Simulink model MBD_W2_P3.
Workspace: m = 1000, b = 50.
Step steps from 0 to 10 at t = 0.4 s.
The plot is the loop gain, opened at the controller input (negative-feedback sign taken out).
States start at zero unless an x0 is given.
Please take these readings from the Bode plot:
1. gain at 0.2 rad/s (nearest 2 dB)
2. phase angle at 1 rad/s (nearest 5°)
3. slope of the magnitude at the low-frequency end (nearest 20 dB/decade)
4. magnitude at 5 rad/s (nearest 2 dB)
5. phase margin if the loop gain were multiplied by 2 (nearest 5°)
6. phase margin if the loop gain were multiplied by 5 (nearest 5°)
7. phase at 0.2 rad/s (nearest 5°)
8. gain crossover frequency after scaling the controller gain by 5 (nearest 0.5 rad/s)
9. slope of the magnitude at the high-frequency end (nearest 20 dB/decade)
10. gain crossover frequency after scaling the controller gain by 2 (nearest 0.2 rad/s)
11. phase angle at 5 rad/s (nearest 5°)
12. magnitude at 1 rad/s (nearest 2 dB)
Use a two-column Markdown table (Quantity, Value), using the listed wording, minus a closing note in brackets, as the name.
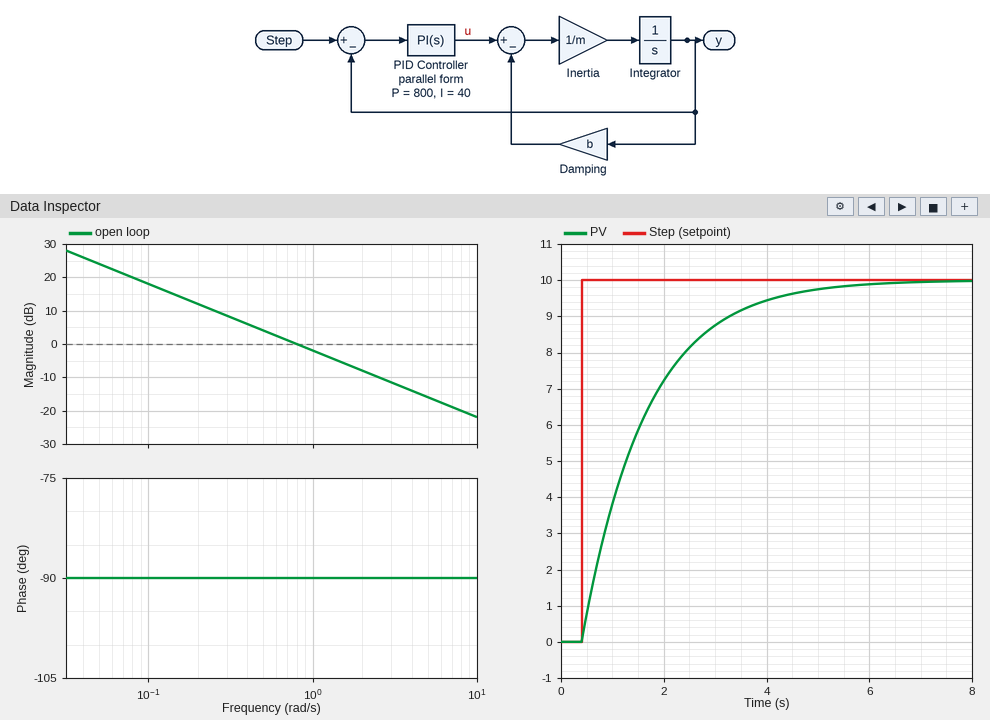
| Quantity | Value |
|---|---|
| gain at 0.2 rad/s | 12 dB |
| phase angle at 1 rad/s | -90° |
| slope of the magnitude at the low-frequency end | -20 dB/decade |
| magnitude at 5 rad/s | -16 dB |
| phase margin if the loop gain were multiplied by 2 | 90° |
| phase margin if the loop gain were multiplied by 5 | 90° |
| phase at 0.2 rad/s | -90° |
| gain crossover frequency after scaling the controller gain by 5 | 4.0 rad/s |
| slope of the magnitude at the high-frequency end | -20 dB/decade |
| gain crossover frequency after scaling the controller gain by 2 | 1.6 rad/s |
| phase angle at 5 rad/s | -90° |
| magnitude at 1 rad/s | -2 dB |
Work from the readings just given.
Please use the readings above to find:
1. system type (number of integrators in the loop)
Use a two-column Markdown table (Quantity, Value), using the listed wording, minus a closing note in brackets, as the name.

| Quantity | Value |
|---|---|
| system type | 1 |
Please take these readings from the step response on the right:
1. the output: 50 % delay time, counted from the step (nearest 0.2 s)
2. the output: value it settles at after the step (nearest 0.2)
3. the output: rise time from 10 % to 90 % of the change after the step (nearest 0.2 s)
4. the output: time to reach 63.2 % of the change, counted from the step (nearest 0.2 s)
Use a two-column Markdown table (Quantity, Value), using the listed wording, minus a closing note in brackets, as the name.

| Quantity | Value |
|---|---|
| the output: 50 % delay time, counted from the step | 0.8 s |
| the output: value it settles at after the step | 10.0 |
| the output: rise time from 10 % to 90 % of the change after the step | 2.8 s |
| the output: time to reach 63.2 % of the change, counted from the step | 1.2 s |
